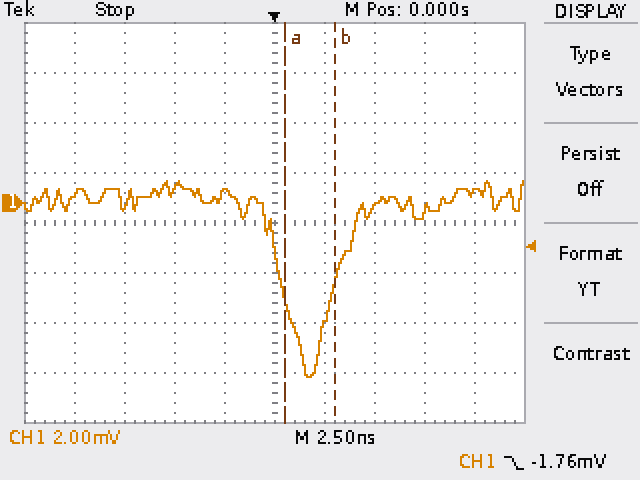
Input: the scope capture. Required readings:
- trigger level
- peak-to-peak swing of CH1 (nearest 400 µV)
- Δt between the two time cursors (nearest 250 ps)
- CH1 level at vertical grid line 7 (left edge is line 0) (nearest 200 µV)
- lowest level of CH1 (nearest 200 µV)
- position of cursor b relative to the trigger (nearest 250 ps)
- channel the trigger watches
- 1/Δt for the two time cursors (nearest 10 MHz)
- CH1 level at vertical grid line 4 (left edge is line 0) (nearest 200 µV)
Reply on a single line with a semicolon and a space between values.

-1.76 mV; 8.0 mV; 2.50 ns; -200 µV; -7.0 mV; +3.00 ns; CH1; 400 MHz; 400 µV
